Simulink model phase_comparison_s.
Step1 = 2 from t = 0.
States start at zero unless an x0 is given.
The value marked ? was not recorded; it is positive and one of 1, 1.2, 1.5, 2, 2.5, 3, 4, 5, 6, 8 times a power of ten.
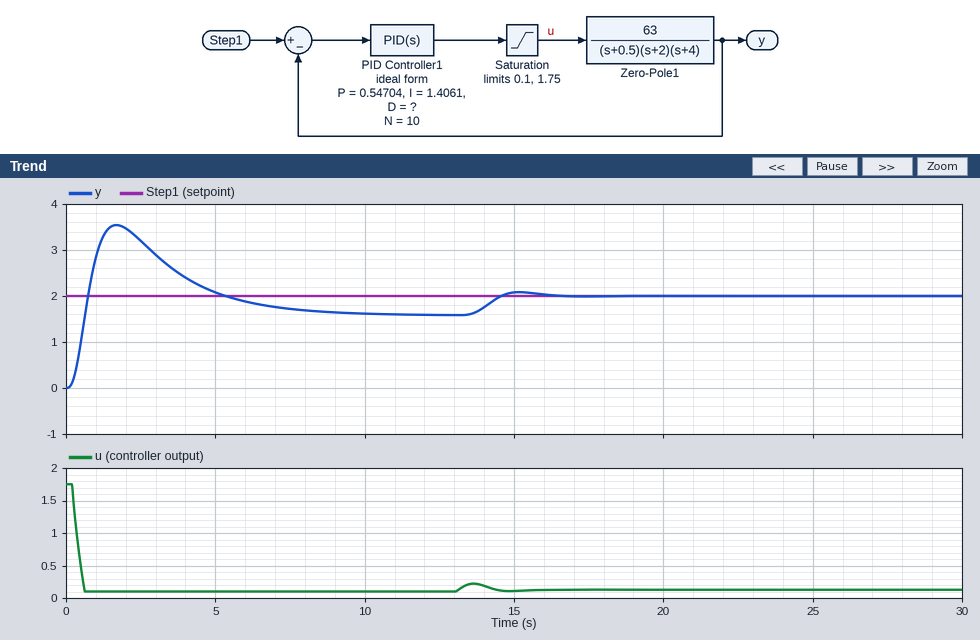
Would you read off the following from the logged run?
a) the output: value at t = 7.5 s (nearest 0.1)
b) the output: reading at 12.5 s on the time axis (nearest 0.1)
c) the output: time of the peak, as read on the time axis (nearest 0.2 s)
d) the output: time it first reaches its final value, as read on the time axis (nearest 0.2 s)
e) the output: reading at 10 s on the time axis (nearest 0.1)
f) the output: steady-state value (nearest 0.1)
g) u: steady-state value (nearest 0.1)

1.7
1.6
1.6 s
0.8 s
1.6
2.0
0.1
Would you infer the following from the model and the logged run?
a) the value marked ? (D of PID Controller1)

0.4
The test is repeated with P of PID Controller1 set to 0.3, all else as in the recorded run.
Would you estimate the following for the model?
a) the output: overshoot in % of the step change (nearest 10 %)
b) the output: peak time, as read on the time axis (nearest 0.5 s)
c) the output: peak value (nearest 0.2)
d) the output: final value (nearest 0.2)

50 %
2.0 s
3.0
2.0
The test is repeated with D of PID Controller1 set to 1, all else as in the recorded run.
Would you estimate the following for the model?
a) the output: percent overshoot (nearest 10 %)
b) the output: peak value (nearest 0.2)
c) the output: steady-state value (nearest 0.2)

50 %
3.0
2.0
